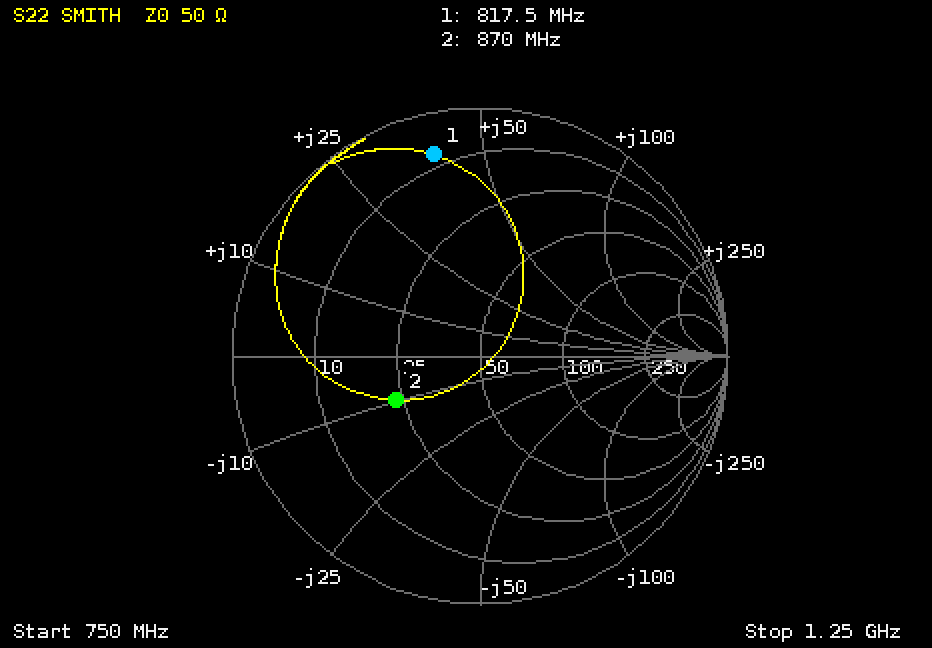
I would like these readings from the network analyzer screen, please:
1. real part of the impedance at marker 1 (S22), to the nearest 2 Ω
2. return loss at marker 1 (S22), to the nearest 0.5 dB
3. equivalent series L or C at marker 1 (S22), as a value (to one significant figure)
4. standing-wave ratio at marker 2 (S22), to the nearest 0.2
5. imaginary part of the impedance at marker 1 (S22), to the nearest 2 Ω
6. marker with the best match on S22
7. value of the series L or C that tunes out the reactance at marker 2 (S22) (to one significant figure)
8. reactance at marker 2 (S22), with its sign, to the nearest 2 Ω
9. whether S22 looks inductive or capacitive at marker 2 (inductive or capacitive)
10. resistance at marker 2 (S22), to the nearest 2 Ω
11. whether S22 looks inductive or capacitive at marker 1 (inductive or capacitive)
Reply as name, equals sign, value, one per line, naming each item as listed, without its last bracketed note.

real part of the impedance at marker 1 (S22), to the nearest 2 Ω = 8 Ω
return loss at marker 1 (S22), to the nearest 0.5 dB = 1.5 dB
equivalent series L or C at marker 1 (S22), as a value = 8 nH
standing-wave ratio at marker 2 (S22), to the nearest 0.2 = 2.2
imaginary part of the impedance at marker 1 (S22), to the nearest 2 Ω = +40 Ω
marker with the best match on S22 = marker 2
value of the series L or C that tunes out the reactance at marker 2 (S22) = 2 nH
reactance at marker 2 (S22), with its sign, to the nearest 2 Ω = -10 Ω
whether S22 looks inductive or capacitive at marker 2 = capacitive
resistance at marker 2 (S22), to the nearest 2 Ω = 24 Ω
whether S22 looks inductive or capacitive at marker 1 = inductive
